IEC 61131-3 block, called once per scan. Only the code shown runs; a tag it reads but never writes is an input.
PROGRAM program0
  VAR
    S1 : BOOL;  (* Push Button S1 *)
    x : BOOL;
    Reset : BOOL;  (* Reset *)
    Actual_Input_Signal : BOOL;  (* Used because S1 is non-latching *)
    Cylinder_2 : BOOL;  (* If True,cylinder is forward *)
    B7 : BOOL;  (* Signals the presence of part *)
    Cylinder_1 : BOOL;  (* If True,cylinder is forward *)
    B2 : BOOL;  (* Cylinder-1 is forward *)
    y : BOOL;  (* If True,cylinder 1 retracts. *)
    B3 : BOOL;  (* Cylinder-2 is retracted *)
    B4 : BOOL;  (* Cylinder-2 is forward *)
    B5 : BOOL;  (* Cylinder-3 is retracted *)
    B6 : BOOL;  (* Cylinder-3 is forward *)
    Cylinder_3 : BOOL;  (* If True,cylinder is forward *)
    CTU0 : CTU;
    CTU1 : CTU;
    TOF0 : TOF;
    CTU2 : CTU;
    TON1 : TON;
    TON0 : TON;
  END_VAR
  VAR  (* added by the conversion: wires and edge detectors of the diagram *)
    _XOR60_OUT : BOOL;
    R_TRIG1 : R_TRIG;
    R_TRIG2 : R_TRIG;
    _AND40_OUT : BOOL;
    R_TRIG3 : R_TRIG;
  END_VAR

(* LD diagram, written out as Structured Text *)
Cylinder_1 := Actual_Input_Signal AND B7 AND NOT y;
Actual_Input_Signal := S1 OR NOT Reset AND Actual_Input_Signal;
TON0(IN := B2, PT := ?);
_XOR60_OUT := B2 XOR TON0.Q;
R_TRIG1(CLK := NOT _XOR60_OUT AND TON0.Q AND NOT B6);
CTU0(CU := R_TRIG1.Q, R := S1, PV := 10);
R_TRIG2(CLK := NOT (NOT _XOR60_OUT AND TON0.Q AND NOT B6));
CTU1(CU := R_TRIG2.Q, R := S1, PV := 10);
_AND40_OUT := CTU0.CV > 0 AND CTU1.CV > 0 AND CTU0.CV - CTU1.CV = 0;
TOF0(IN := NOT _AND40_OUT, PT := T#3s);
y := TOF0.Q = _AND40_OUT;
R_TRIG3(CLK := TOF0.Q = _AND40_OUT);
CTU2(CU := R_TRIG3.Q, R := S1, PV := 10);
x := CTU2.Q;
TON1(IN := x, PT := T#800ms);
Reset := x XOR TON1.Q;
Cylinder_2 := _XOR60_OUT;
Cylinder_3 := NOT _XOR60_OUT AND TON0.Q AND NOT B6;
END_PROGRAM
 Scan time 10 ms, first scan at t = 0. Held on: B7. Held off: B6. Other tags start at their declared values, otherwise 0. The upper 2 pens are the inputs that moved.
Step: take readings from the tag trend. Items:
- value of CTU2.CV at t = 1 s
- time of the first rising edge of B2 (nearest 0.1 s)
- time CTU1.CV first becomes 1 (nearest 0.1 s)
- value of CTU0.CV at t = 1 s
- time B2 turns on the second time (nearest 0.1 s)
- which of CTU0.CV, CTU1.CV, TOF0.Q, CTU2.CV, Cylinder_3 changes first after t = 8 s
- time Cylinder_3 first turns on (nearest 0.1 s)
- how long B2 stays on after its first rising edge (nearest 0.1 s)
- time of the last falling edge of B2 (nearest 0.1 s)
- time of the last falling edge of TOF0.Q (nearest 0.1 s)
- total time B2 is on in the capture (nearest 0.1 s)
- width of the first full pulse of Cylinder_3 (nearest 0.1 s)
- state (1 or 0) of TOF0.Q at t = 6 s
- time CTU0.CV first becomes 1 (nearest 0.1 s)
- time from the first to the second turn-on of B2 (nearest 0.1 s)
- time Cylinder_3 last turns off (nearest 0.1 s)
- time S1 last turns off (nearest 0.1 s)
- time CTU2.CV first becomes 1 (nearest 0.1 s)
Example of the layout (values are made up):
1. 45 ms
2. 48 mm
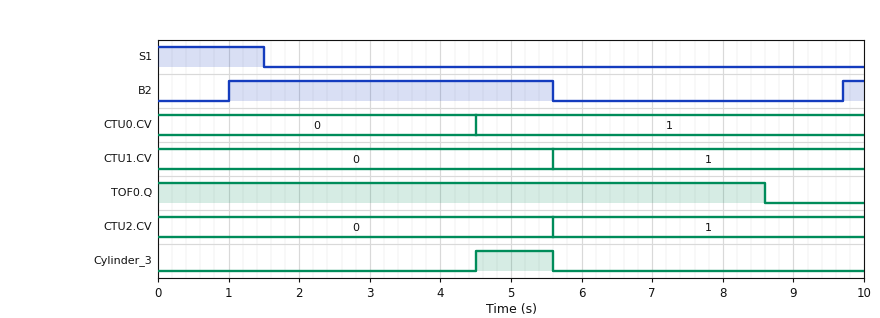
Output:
1. 0
2. 1.0 s
3. 5.6 s
4. 0
5. 9.7 s
6. TOF0.Q
7. 4.5 s
8. 4.6 s
9. 5.6 s
10. 8.6 s
11. 4.9 s
12. 1.1 s
13. 1
14. 4.5 s
15. 8.7 s
16. 5.6 s
17. 1.5 s
18. 5.6 s
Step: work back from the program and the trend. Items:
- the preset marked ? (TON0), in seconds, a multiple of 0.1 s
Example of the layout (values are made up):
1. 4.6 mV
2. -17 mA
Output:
1. 3.5 s
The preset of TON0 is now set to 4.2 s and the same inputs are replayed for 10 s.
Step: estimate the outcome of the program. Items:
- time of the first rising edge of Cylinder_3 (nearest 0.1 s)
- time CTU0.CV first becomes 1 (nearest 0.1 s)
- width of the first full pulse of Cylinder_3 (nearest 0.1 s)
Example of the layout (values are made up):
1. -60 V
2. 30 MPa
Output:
1. 5.2 s
2. 5.2 s
3. 0.4 s
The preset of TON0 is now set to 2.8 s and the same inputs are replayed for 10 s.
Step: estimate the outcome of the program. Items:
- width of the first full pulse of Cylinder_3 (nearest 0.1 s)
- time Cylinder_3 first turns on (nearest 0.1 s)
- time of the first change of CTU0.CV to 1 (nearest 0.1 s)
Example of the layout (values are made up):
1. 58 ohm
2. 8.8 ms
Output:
1. 1.8 s
2. 3.8 s
3. 3.8 s
